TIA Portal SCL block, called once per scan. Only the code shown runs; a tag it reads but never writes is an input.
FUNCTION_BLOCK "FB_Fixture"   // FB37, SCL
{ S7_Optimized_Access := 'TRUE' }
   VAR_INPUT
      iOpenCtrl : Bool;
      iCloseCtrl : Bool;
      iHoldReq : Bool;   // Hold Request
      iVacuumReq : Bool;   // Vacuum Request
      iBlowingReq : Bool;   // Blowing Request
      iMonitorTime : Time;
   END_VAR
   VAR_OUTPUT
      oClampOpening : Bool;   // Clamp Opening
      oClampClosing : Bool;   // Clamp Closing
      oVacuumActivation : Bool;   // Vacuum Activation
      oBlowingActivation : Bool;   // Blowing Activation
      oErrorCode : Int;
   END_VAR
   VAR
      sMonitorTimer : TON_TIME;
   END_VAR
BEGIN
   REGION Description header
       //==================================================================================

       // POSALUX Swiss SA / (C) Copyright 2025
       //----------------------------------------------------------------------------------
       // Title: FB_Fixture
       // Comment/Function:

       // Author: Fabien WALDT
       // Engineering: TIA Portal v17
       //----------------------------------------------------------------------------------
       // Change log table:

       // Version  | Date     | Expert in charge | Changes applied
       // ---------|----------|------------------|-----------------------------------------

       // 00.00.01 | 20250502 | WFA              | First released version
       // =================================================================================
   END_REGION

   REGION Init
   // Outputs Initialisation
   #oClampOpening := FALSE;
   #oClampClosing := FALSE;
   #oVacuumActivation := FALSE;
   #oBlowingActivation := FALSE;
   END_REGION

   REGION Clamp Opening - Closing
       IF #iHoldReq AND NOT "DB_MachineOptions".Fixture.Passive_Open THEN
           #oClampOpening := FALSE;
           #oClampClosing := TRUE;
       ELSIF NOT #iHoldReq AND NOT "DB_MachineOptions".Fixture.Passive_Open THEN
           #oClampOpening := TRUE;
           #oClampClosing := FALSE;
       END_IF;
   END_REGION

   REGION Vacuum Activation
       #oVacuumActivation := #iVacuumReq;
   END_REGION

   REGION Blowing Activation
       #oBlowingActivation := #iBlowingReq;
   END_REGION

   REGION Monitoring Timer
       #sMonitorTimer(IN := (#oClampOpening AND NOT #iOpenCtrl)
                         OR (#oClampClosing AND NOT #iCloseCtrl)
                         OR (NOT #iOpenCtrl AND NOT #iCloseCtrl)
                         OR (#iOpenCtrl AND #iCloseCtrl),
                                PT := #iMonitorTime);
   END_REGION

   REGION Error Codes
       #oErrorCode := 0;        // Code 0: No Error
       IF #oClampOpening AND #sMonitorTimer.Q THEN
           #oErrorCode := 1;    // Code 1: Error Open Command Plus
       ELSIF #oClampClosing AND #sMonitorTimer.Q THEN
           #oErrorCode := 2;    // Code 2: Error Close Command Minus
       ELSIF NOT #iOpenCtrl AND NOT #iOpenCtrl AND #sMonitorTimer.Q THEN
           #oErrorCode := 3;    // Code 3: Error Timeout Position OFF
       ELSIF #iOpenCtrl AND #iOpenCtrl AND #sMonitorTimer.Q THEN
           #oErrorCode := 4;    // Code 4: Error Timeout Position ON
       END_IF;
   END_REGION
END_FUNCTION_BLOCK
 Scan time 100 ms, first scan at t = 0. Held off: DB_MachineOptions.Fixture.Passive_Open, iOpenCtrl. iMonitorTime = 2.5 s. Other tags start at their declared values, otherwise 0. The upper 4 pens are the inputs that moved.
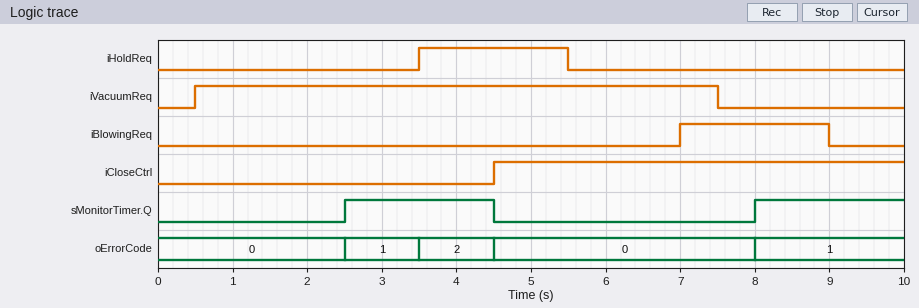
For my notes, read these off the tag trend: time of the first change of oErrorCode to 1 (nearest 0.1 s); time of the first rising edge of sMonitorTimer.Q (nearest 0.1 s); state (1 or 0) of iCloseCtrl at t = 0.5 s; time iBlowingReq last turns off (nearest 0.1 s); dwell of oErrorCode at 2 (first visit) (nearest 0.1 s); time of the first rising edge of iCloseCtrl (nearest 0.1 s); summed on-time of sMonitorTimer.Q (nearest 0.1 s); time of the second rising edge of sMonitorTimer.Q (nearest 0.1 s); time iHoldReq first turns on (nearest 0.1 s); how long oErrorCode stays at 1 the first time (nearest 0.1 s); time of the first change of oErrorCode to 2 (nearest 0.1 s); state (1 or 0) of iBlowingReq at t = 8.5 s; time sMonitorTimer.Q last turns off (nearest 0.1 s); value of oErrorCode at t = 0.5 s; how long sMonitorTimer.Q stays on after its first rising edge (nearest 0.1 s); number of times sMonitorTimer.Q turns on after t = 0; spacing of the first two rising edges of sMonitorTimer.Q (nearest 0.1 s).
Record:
2.5 s
2.5 s
0
9.0 s
1.0 s
4.5 s
4.0 s
8.0 s
3.5 s
1.0 s
3.5 s
1
4.5 s
0
2.0 s
2
5.5 s
